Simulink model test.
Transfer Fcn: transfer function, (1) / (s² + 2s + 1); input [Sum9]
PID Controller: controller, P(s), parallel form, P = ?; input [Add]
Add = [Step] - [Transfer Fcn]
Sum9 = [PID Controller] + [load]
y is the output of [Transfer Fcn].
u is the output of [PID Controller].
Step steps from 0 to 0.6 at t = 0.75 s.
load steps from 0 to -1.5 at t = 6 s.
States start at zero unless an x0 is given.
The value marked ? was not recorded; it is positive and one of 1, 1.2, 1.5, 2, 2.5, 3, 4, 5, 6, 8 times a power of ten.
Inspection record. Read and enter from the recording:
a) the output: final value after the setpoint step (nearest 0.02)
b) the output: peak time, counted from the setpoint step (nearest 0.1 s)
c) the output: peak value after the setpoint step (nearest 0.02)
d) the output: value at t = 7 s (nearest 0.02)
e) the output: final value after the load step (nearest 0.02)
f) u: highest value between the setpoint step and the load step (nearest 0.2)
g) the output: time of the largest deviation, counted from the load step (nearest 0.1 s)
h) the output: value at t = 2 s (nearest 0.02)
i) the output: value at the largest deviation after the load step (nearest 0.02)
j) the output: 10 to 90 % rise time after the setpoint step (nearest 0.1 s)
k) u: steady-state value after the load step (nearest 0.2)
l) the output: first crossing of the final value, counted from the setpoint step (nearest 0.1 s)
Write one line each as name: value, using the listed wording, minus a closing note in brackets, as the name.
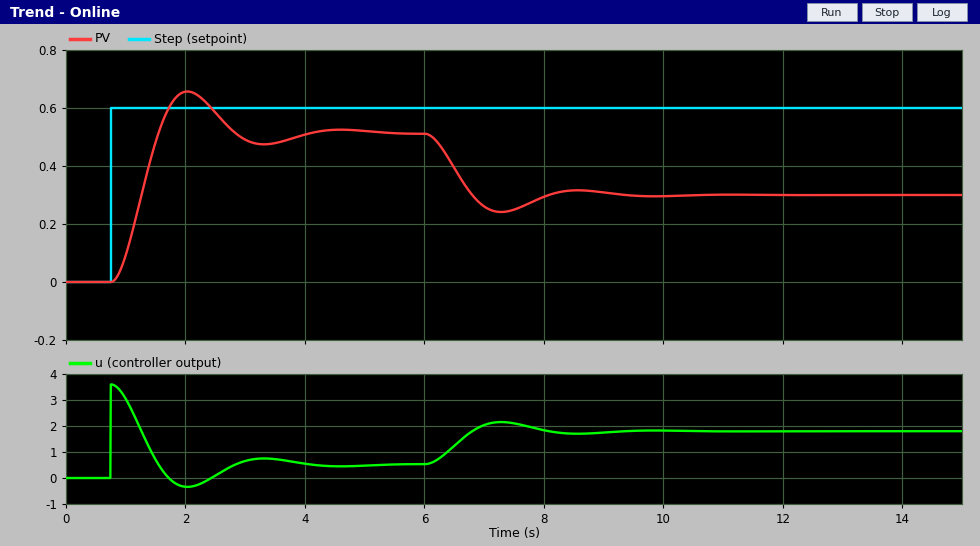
the output: final value after the setpoint step: 0.52
the output: peak time, counted from the setpoint step: 1.3 s
the output: peak value after the setpoint step: 0.66
the output: value at t = 7 s: 0.26
the output: final value after the load step: 0.30
u: highest value between the setpoint step and the load step: 3.6
the output: time of the largest deviation, counted from the load step: 1.3 s
the output: value at t = 2 s: 0.66
the output: value at the largest deviation after the load step: 0.24
the output: 10 to 90 % rise time after the setpoint step: 0.5 s
u: steady-state value after the load step: 1.8
the output: first crossing of the final value, counted from the setpoint step: 0.8 s
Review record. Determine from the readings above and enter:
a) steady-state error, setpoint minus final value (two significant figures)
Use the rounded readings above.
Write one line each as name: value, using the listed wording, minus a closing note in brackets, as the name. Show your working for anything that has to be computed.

steady-state error, setpoint minus final value: 0.6 - 0.52 = 0.080
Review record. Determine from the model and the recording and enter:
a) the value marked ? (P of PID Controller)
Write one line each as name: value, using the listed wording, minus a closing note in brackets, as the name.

the value marked ?: 6
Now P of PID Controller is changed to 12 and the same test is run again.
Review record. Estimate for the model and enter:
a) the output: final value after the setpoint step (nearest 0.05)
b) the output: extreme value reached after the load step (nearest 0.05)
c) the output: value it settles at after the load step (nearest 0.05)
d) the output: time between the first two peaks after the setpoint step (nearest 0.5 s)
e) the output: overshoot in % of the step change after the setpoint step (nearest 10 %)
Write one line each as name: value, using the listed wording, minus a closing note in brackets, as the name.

the output: final value after the setpoint step: 0.55
the output: extreme value reached after the load step: 0.40
the output: value it settles at after the load step: 0.45
the output: time between the first two peaks after the setpoint step: 2.0 s
the output: overshoot in % of the step change after the setpoint step: 40 %
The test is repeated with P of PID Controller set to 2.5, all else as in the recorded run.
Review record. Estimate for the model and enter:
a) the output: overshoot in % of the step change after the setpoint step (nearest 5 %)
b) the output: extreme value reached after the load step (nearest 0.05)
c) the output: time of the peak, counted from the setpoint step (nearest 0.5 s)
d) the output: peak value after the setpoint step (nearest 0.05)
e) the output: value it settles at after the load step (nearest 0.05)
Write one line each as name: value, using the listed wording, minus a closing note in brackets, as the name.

the output: overshoot in % of the step change after the setpoint step: 15 %
the output: extreme value reached after the load step: -0.05
the output: time of the peak, counted from the setpoint step: 2.0 s
the output: peak value after the setpoint step: 0.50
the output: value it settles at after the load step: 0.00
